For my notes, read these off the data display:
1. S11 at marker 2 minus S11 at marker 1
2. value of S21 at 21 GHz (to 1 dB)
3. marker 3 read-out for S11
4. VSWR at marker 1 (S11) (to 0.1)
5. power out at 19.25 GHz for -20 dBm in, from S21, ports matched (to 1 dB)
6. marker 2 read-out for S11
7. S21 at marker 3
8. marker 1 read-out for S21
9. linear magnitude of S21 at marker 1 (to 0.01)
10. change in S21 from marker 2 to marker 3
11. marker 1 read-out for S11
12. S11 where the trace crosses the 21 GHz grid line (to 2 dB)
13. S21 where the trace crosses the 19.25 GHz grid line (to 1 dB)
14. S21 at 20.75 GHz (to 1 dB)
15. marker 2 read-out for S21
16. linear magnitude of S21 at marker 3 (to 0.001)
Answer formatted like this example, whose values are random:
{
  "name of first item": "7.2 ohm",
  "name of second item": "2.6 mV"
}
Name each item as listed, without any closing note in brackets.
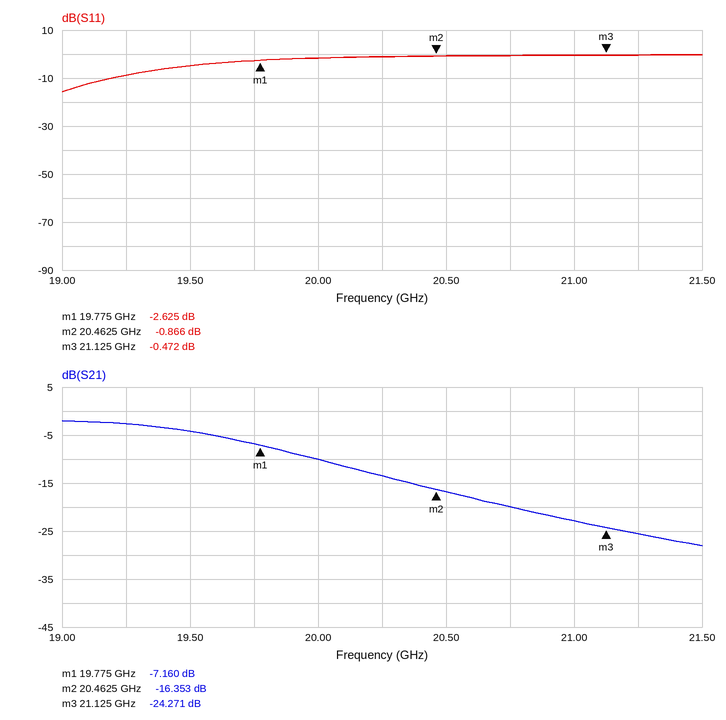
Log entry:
{
  "S11 at marker 2 minus S11 at marker 1": "1.759 dB",
  "value of S21 at 21 GHz": "-23 dB",
  "marker 3 read-out for S11": "-0.472 dB",
  "VSWR at marker 1 (S11)": "6.7",
  "power out at 19.25 GHz for -20 dBm in, from S21, ports matched": "-23 dBm",
  "marker 2 read-out for S11": "-0.866 dB",
  "S21 at marker 3": "-24.271 dB",
  "marker 1 read-out for S21": "-7.160 dB",
  "linear magnitude of S21 at marker 1": "0.44",
  "change in S21 from marker 2 to marker 3": "-7.918 dB",
  "marker 1 read-out for S11": "-2.625 dB",
  "S11 where the trace crosses the 21 GHz grid line": "0 dB",
  "S21 where the trace crosses the 19.25 GHz grid line": "-3 dB",
  "S21 at 20.75 GHz": "-20 dB",
  "marker 2 read-out for S21": "-16.353 dB",
  "linear magnitude of S21 at marker 3": "0.061"
}
